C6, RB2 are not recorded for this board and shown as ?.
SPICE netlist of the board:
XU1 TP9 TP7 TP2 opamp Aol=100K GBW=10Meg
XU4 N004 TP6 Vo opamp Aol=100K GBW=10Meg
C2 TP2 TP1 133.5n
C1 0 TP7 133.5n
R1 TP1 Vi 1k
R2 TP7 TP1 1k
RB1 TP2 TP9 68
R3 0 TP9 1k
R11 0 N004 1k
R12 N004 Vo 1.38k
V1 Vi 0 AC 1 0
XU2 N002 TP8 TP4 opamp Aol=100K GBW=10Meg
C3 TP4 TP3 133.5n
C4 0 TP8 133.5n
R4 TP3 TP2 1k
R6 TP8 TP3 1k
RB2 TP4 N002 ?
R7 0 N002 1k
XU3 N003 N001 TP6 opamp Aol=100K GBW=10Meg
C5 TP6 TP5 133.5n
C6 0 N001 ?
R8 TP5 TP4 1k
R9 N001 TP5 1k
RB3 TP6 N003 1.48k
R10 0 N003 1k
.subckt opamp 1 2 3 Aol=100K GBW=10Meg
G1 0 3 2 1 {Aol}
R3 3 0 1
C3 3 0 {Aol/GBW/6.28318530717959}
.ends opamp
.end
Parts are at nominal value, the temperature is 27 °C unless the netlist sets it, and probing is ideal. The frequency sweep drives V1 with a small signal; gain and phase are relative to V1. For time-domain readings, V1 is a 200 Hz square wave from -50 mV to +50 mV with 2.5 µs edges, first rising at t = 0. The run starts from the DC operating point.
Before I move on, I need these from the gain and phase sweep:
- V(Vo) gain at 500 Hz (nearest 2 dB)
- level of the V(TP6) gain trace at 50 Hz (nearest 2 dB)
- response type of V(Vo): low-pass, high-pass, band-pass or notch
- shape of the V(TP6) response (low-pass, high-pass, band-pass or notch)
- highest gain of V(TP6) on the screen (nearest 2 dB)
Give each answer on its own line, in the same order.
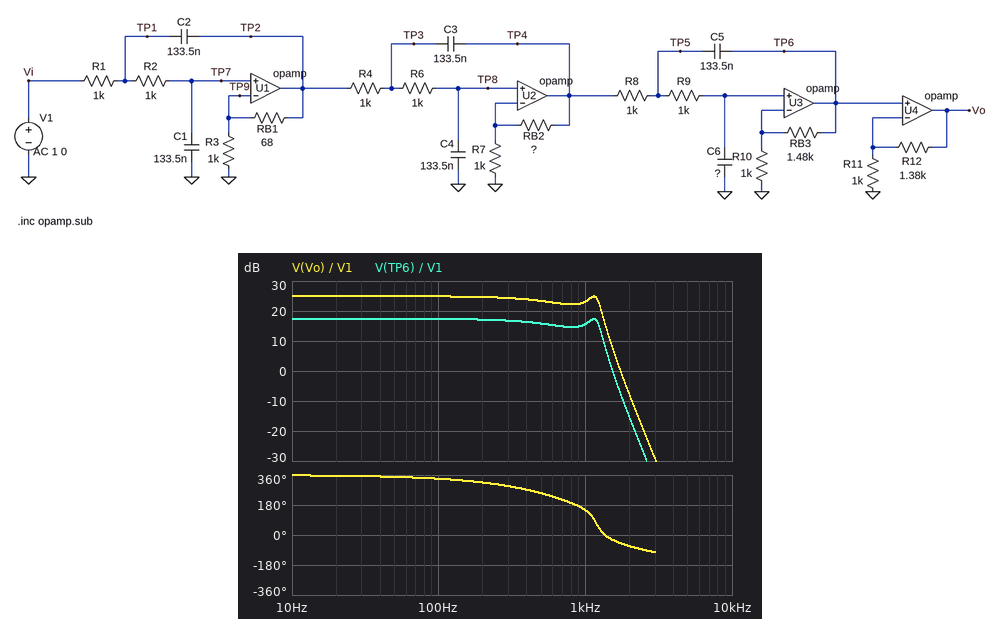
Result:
24 dB
18 dB
low-pass
low-pass
18 dB
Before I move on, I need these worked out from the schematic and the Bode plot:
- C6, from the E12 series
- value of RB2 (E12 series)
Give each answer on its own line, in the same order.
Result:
270 nF
1.8 kΩ
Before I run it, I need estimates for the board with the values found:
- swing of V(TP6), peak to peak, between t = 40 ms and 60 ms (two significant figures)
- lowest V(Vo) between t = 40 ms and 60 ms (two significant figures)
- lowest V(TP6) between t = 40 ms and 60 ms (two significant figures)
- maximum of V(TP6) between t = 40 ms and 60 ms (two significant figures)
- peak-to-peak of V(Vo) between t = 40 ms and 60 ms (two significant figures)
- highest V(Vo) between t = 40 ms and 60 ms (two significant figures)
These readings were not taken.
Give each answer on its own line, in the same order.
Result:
820 mV
-980 mV
-410 mV
410 mV
2.0 V
980 mV
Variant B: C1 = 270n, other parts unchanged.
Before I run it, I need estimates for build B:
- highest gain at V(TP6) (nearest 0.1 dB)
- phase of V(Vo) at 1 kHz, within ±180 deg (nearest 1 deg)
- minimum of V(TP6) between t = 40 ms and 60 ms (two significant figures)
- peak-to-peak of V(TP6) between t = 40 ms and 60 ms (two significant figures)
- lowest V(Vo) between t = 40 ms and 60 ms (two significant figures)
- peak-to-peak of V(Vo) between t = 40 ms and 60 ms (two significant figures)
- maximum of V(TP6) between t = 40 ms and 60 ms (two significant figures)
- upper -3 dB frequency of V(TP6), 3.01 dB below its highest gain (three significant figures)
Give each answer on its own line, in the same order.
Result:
17.4 dB
132 deg
-370 mV
750 mV
-890 mV
1.8 V
370 mV
329 Hz
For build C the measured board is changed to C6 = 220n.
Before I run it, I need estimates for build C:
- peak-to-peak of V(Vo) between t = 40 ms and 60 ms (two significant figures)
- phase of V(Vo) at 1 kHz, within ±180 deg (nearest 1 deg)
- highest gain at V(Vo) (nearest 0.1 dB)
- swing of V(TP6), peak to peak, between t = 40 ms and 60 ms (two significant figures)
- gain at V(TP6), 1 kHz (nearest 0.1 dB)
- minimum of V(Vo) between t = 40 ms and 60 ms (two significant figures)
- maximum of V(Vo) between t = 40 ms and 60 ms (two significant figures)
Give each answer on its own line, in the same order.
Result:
2.4 V
155 deg
28.0 dB
990 mV
18.7 dB
-1.2 V
1.2 V
